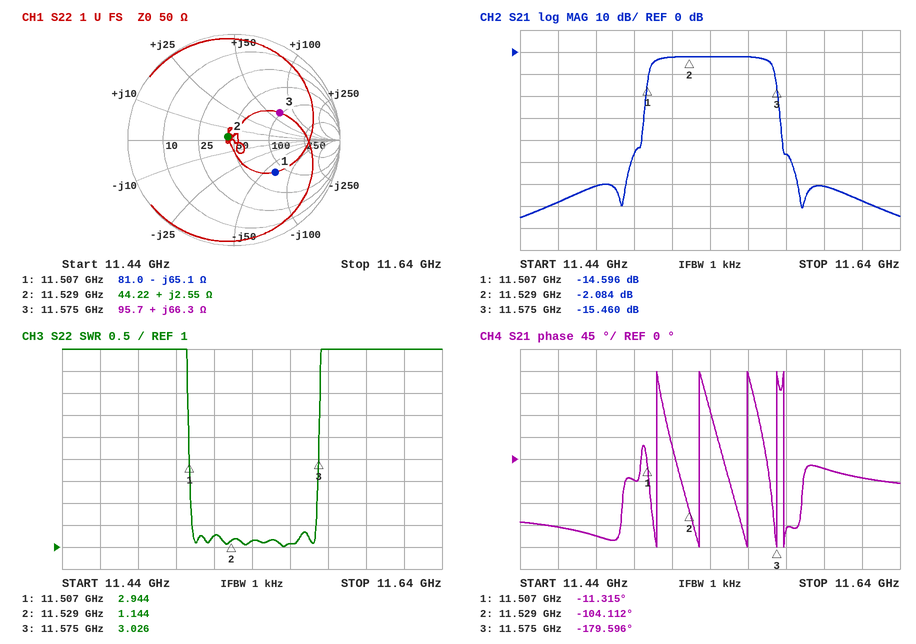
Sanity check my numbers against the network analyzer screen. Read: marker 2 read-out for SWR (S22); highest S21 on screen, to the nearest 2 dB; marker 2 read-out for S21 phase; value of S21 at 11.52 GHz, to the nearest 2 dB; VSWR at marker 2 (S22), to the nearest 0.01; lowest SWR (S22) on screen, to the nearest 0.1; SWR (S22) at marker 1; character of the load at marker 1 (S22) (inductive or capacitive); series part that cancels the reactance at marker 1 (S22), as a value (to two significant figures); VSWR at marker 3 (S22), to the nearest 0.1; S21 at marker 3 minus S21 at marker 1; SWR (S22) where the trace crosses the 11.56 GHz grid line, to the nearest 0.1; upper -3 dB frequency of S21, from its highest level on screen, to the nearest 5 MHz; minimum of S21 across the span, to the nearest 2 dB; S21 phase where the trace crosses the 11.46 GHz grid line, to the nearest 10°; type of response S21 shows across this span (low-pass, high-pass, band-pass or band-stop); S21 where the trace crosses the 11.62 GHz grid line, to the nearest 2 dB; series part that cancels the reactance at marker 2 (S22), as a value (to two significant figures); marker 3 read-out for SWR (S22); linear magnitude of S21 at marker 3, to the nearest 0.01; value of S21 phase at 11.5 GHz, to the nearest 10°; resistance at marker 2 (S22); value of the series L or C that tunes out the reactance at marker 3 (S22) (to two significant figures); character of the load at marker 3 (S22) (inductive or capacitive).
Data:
1.144
-2 dB
-104.112°
-2 dB
1.14
1.0
2.944
capacitive
900 pH
3.0
-0.864 dB
1.1
11.570 GHz
-76 dB
-140°
band-pass
-68 dB
5.4 pF
3.026
0.17
-40°
44.22 Ω
210 fF
inductive
